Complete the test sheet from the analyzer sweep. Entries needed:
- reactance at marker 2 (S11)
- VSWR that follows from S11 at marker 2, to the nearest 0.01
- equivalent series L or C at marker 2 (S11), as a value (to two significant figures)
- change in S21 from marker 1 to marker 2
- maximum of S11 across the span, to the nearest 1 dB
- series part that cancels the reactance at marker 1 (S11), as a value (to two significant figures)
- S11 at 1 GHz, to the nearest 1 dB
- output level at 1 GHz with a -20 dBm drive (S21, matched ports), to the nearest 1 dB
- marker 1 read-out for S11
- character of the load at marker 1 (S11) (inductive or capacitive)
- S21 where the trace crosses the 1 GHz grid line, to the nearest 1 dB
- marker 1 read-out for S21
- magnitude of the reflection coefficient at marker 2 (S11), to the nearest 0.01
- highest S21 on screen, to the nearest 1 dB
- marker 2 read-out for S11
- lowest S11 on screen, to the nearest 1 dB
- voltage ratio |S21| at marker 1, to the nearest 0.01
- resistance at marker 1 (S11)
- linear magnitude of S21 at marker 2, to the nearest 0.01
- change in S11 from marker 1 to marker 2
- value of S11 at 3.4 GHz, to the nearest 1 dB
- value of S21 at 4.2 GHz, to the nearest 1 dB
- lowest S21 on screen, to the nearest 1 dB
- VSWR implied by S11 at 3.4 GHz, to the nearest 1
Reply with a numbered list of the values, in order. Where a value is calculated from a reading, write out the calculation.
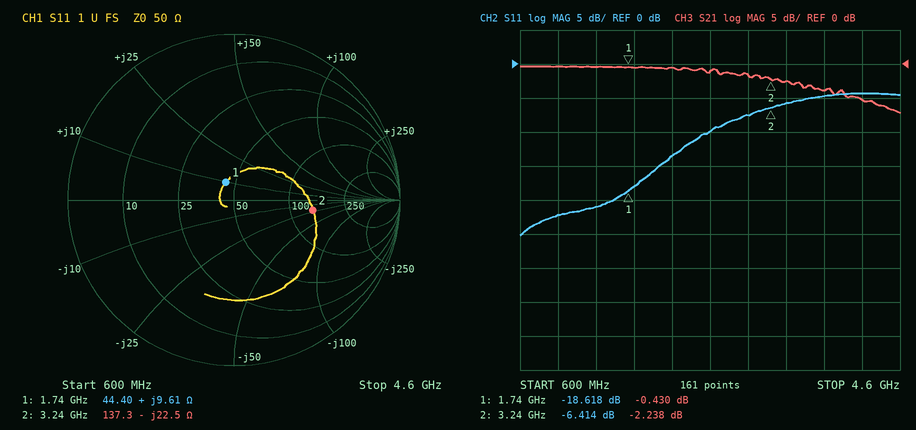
1. -22.5 Ω
2. (1 + 0.4779)/(1 − 0.4779) ≈ 2.83
3. C = 1/(2π × 3.24 GHz × 22.5 Ω) ≈ 2.2 pF
4. -2.238 − (-0.43) = -1.808 dB
5. -4 dB
6. C = 1/(2π × 1.74 GHz × 9.61 Ω) ≈ 9.5 pF
7. -22 dB
8. -20 dBm + (0 dB) = -20 dBm
9. -18.618 dB
10. inductive
11. 0 dB
12. -0.430 dB
13. 0.48
14. 0 dB
15. -6.414 dB
16. -25 dB
17. 10^(-0.43/20) ≈ 0.95
18. 44.40 Ω
19. 10^(-2.238/20) ≈ 0.77
20. -6.414 − (-18.618) = 12.204 dB
21. -6 dB
22. -5 dB
23. -7 dB
24. |Γ| = 10^(-6/20) = 0.5012; VSWR = (1 + 0.5012)/(1 − 0.5012) ≈ 3
